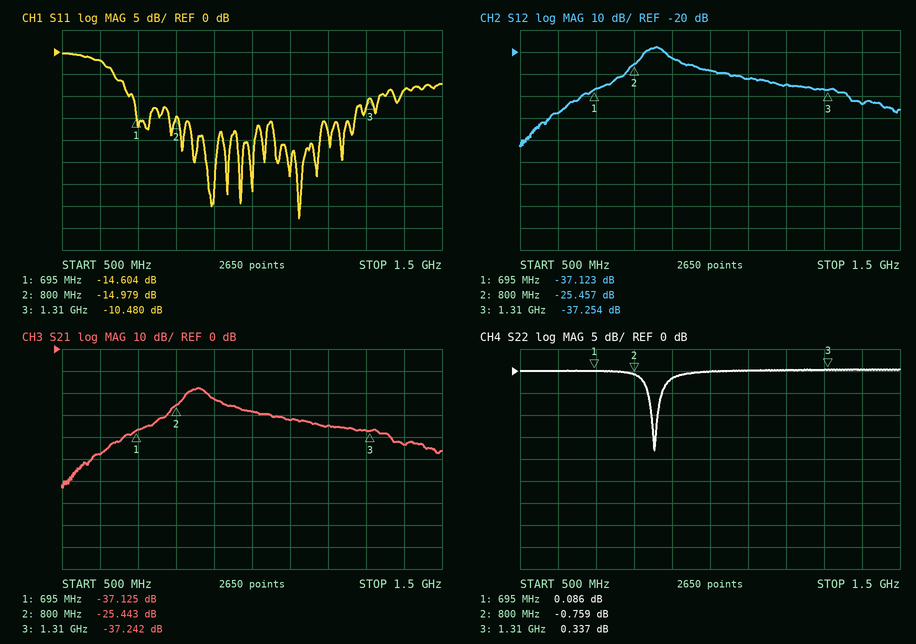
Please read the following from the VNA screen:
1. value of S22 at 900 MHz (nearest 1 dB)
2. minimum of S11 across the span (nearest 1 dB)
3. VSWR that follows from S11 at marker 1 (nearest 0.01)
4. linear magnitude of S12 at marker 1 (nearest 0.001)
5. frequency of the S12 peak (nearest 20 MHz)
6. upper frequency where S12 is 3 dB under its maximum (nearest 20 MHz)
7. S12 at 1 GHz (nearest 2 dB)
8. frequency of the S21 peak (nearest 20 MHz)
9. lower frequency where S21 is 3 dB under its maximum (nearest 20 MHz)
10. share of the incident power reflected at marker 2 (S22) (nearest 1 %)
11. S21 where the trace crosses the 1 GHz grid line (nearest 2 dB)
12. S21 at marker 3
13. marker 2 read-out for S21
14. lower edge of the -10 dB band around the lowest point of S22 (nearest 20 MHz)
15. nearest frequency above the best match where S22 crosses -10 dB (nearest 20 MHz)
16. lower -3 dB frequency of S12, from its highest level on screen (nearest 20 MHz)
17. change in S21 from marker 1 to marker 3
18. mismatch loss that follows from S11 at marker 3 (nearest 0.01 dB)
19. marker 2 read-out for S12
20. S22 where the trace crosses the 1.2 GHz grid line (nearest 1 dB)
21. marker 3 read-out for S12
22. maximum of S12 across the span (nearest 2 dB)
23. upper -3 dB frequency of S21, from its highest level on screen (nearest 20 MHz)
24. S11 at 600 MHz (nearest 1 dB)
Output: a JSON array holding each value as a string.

["-2 dB", "-38 dB", "1.46", "0.014", "860 MHz", "880 MHz", "-28 dB", "860 MHz", "820 MHz", "84 %", "-28 dB", "-37.242 dB", "-25.443 dB", "840 MHz", "860 MHz", "820 MHz", "-0.117 dB", "0.41 dB", "-25.457 dB", "0 dB", "-37.254 dB", "-18 dB", "880 MHz", "-2 dB"]
